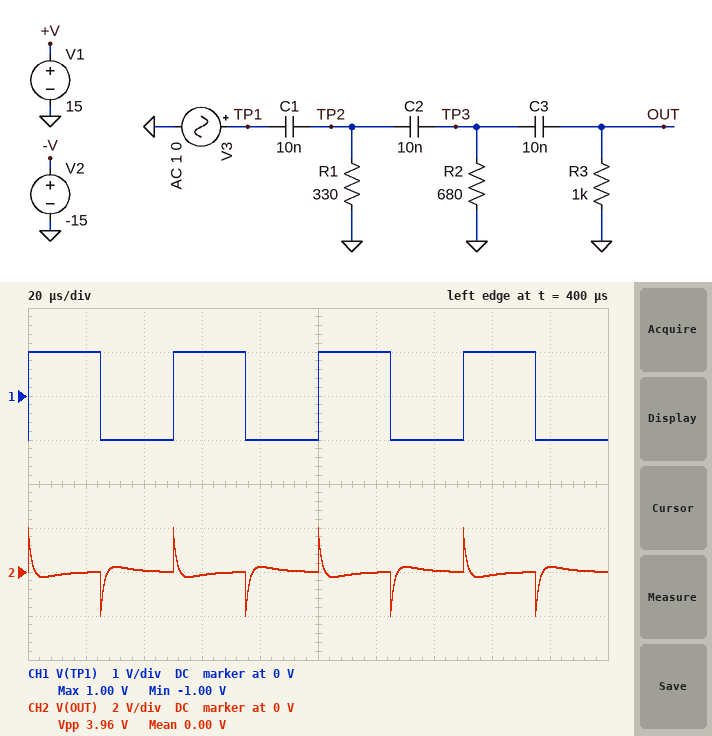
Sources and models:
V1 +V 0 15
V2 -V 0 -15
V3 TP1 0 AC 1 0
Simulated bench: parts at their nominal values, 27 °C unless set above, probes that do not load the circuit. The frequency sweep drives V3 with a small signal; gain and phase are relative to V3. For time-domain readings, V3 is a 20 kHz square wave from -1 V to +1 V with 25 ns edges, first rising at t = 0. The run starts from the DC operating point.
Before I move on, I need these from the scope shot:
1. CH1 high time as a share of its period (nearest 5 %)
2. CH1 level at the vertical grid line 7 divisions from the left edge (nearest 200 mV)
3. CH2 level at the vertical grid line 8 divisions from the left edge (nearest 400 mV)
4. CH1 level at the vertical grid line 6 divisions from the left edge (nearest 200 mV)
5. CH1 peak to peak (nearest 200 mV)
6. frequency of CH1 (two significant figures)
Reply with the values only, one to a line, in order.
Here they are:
50 %
-1.0 V
0 V
1.0 V
2.0 V
20 kHz
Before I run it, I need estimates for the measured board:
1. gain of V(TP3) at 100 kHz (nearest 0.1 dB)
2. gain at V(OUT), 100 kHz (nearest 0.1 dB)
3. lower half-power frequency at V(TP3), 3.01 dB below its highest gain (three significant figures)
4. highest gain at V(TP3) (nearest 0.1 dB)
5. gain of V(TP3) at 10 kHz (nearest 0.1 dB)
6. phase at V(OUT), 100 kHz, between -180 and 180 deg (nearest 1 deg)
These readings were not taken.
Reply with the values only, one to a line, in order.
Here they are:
-3.7 dB
-3.8 dB
116 kHz
0 dB
-25.0 dB
65 deg
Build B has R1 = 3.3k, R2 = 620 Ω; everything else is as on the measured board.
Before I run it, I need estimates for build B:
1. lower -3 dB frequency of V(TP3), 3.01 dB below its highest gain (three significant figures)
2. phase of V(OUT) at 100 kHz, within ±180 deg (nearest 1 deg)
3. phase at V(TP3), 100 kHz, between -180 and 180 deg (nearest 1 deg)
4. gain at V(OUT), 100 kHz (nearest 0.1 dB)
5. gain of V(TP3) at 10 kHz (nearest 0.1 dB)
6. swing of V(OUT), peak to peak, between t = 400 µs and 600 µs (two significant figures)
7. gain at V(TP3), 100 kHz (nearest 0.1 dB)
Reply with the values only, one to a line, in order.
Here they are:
90.5 kHz
49 deg
40 deg
-2.7 dB
-16.8 dB
4.1 V
-2.6 dB
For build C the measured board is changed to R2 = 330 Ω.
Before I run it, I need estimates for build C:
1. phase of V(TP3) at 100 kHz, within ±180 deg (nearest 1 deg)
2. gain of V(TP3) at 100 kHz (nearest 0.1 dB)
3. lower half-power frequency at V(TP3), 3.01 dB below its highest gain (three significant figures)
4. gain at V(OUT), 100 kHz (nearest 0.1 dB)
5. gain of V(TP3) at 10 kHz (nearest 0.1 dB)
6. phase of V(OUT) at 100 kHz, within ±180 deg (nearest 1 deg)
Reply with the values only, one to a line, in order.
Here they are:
67 deg
-5.7 dB
162 kHz
-5.8 dB
-29.5 dB
76 deg
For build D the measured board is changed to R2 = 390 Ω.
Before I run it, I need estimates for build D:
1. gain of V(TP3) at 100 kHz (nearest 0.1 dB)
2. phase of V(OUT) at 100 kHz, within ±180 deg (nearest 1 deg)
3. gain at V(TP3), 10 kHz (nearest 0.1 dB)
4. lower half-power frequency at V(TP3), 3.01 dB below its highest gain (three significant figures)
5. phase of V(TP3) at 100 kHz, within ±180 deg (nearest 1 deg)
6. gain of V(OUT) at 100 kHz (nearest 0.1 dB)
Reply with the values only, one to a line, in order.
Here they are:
-5.1 dB
73 deg
-28.3 dB
148 kHz
64 deg
-5.2 dB
